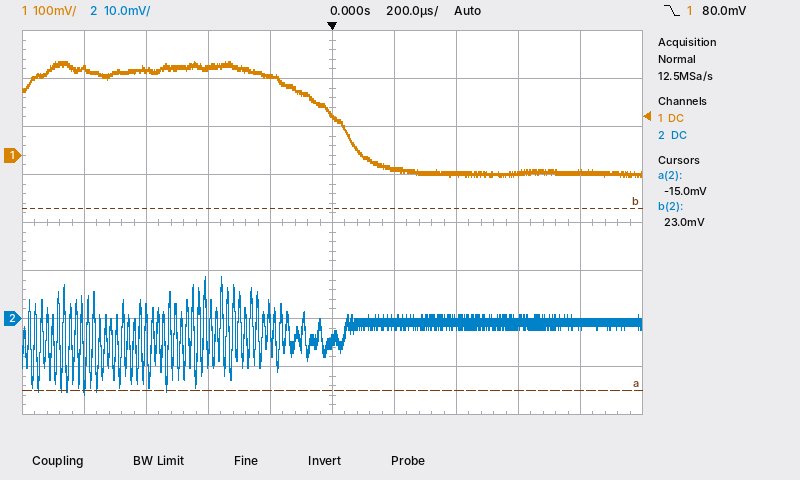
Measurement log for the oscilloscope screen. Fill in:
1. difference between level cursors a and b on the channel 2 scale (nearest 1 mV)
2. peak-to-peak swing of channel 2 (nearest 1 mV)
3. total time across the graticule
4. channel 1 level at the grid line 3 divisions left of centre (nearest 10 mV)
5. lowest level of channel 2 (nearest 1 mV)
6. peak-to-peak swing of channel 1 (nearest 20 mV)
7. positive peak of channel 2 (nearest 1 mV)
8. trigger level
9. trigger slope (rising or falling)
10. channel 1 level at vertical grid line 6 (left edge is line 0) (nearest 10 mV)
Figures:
38 mV
25 mV
2 ms
180 mV
-16 mV
240 mV
9 mV
80.0 mV
falling
-30 mV
